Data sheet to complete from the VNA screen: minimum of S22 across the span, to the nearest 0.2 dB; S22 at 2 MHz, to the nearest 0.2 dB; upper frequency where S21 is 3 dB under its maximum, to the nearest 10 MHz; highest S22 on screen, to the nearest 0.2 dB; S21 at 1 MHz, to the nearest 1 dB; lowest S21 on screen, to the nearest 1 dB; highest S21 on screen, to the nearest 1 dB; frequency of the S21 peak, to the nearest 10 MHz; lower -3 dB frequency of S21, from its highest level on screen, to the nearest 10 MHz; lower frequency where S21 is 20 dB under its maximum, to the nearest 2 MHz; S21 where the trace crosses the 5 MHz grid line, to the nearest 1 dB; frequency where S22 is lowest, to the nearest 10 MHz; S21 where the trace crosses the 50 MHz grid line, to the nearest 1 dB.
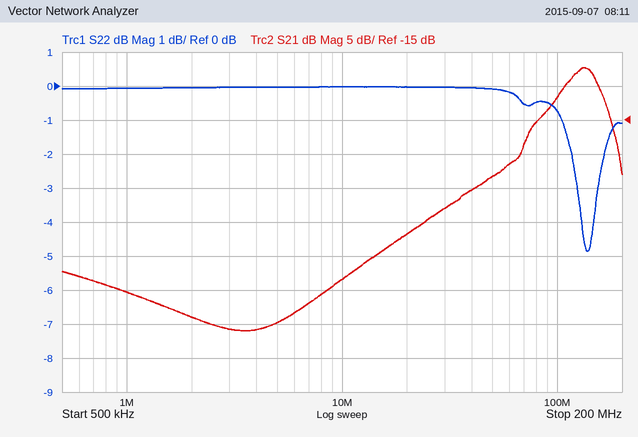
-4.8 dB
0.0 dB
160 MHz
0.0 dB
-40 dB
-46 dB
-7 dB
130 MHz
110 MHz
32 MHz
-45 dB
140 MHz
-23 dB
